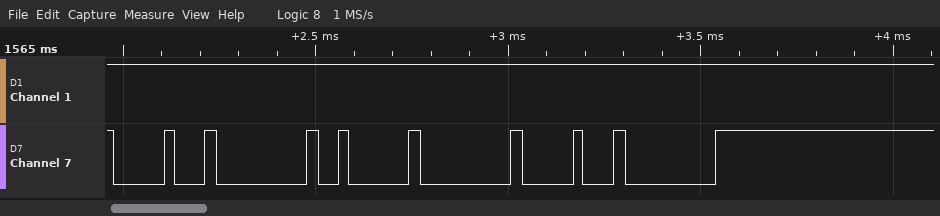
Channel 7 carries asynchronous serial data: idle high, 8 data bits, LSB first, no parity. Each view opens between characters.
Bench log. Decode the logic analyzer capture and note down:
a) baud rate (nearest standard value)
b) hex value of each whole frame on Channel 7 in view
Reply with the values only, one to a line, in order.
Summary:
38400 baud
10, 00, 02, 00, 10, 00
